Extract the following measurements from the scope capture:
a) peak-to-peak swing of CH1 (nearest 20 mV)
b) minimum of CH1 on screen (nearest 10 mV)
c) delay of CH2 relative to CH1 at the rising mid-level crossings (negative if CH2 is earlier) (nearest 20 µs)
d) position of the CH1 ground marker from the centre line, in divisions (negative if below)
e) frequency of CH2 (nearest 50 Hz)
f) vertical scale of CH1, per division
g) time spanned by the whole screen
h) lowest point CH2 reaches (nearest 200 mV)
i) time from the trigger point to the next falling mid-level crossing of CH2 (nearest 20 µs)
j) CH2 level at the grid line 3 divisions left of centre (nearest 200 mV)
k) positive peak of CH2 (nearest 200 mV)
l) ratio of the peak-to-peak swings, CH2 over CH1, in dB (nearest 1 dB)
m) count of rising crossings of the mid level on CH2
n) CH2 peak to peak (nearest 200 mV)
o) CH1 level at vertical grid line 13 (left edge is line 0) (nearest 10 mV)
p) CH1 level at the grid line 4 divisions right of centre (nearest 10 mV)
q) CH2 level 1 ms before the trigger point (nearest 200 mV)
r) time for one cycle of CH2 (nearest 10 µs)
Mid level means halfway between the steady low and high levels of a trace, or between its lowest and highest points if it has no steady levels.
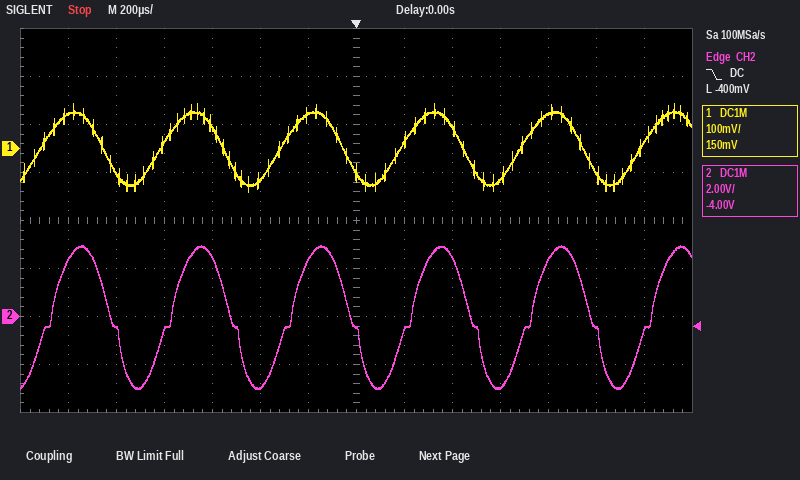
180 mV
-90 mV
+40 µs
+1.5 div
2.00 kHz
100 mV
2.8 ms
-3.0 V
480 µs
2.4 V
3.0 V
30 dB
6
6.0 V
10 mV
70 mV
-400 mV
500 µs
